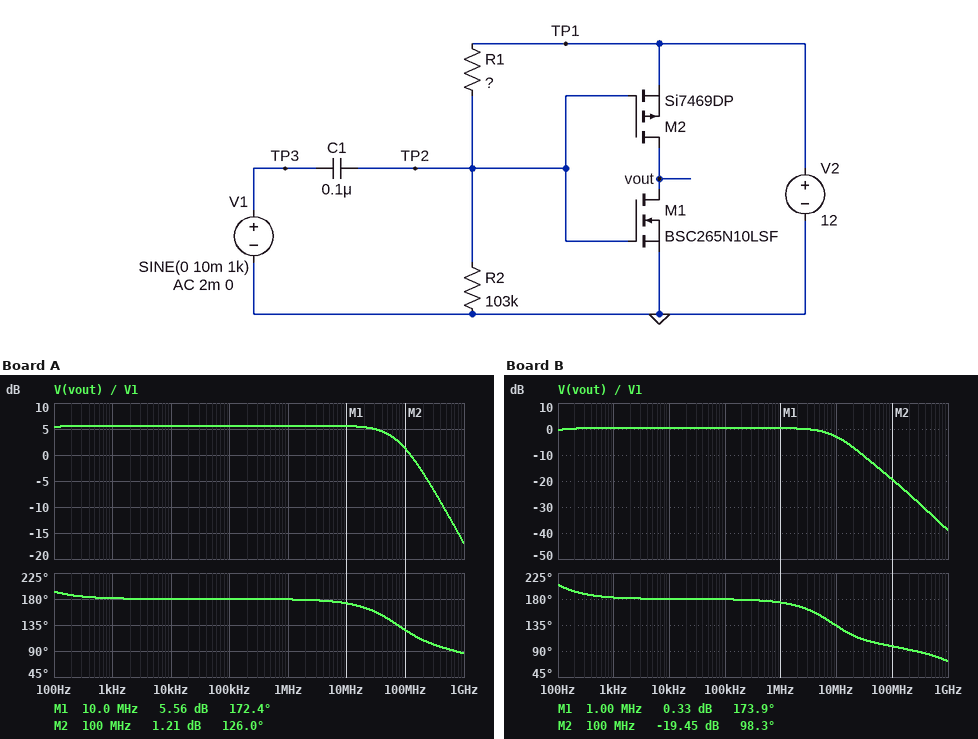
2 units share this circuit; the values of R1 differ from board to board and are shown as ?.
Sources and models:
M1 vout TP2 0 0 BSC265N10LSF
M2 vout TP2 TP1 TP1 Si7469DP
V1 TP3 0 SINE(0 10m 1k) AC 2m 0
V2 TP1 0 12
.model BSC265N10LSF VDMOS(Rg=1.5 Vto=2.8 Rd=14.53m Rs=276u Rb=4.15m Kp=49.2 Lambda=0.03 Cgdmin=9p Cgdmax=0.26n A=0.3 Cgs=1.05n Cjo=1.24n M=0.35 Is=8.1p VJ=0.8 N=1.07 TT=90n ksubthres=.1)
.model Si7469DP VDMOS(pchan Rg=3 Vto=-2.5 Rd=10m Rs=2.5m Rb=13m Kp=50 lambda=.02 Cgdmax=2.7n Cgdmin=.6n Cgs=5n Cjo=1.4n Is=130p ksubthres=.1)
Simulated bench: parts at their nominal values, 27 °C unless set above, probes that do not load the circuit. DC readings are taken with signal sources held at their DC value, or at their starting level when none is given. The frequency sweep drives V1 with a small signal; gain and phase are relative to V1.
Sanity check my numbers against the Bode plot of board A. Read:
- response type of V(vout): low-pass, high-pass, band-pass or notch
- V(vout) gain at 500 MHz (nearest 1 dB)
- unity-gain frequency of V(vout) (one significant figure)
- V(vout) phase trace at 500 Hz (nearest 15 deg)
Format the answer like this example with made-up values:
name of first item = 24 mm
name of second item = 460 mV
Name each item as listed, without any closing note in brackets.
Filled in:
response type of V(vout): low-pass, high-pass, band-pass or notch = low-pass
V(vout) gain at 500 MHz = -11 dB
unity-gain frequency of V(vout) = 100 MHz
V(vout) phase trace at 500 Hz = 180 deg
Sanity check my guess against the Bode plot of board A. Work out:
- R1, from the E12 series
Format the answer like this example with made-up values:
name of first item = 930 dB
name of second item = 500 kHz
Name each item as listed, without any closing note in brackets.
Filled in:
R1, from the E12 series = 150 kΩ
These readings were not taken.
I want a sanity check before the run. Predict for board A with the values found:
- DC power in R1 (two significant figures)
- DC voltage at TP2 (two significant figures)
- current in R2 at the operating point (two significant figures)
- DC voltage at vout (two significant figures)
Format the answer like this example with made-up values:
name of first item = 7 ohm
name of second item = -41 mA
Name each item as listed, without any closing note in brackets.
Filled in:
DC power in R1 = 340 µW
DC voltage at TP2 = 4.9 V
current in R2 at the operating point = 47 µA
DC voltage at vout = 9.8 V
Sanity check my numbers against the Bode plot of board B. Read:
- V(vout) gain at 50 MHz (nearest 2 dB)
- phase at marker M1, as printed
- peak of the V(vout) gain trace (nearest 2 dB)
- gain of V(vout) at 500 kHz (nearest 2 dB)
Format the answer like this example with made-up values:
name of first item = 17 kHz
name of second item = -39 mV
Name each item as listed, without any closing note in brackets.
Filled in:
V(vout) gain at 50 MHz = -14 dB
phase at marker M1, as printed = 173.9 deg
peak of the V(vout) gain trace = 0 dB
gain of V(vout) at 500 kHz = 0 dB
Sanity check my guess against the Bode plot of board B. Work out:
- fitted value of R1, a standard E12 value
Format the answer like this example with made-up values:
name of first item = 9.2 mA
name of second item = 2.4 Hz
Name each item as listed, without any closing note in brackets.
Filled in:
fitted value of R1, a standard E12 value = 47 kΩ
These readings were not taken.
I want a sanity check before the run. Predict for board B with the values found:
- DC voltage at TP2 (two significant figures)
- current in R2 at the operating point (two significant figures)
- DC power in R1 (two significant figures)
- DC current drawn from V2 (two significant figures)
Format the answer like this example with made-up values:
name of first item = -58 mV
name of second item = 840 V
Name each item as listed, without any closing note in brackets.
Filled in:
DC voltage at TP2 = 8.2 V
current in R2 at the operating point = 80 µA
DC power in R1 = 300 µW
DC current drawn from V2 = 41 A
